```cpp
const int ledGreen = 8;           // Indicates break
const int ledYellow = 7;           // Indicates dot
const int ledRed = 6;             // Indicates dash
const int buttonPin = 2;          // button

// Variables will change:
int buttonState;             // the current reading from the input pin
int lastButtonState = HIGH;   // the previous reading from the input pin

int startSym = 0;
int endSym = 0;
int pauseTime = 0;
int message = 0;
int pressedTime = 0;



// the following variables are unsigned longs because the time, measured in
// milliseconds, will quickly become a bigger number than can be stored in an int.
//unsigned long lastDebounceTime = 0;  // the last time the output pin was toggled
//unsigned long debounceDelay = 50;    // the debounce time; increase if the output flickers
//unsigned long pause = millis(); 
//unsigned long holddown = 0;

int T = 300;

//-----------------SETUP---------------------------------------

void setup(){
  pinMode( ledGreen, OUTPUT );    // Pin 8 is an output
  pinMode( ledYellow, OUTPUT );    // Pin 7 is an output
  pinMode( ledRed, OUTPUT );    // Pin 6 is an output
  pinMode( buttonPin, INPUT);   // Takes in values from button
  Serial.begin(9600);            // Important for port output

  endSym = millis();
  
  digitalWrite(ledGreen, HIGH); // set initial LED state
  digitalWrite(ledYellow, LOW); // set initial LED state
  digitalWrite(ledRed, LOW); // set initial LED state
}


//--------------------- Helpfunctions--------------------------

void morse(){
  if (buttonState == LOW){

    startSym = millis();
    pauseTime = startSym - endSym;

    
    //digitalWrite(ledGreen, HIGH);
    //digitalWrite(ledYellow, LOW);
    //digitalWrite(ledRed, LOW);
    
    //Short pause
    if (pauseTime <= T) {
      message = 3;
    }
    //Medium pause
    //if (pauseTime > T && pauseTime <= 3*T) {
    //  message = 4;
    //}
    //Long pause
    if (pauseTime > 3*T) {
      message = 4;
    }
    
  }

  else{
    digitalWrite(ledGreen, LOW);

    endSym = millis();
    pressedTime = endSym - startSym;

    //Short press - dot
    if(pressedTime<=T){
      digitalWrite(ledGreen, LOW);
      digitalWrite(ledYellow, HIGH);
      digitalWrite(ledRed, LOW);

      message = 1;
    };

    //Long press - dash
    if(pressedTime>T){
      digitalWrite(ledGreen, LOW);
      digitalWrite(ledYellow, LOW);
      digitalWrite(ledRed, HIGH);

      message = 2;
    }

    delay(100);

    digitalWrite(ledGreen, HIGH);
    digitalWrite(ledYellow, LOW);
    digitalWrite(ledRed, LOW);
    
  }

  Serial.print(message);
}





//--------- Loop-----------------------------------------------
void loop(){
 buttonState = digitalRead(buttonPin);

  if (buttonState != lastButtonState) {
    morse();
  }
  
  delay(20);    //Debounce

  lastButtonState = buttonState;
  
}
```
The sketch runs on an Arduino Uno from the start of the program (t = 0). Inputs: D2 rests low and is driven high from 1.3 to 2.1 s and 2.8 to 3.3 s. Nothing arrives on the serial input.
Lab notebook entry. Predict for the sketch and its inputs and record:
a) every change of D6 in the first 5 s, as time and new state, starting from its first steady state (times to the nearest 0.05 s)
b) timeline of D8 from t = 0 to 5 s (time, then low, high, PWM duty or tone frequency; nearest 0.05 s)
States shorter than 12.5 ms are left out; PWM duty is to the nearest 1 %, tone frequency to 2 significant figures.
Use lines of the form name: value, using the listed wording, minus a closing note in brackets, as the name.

every change of D6 in the first 5 s, as time and new state, starting from its first steady state: 0 s low; 1.3 s high; 1.4 s low; 2.8 s high; 2.9 s low
timeline of D8 from t = 0 to 5 s: 0 s high; 1.3 s low; 1.4 s high; 2.8 s low; 2.9 s high
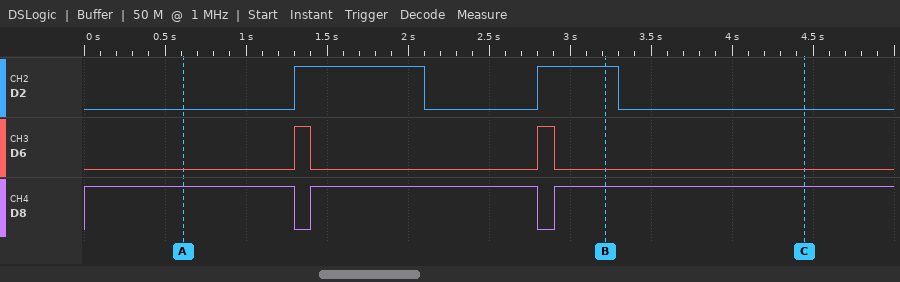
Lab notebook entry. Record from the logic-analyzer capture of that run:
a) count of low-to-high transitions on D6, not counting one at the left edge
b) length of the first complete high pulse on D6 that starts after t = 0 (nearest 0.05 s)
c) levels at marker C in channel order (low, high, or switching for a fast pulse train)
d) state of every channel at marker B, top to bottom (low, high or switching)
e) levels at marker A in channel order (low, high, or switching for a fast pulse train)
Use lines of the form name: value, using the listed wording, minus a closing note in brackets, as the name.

count of low-to-high transitions on D6, not counting one at the left edge: 2
length of the first complete high pulse on D6 that starts after t = 0: 0.10 s
levels at marker C in channel order: D2 low, D6 low, D8 high
state of every channel at marker B, top to bottom: D2 high, D6 low, D8 high
levels at marker A in channel order: D2 low, D6 low, D8 high
